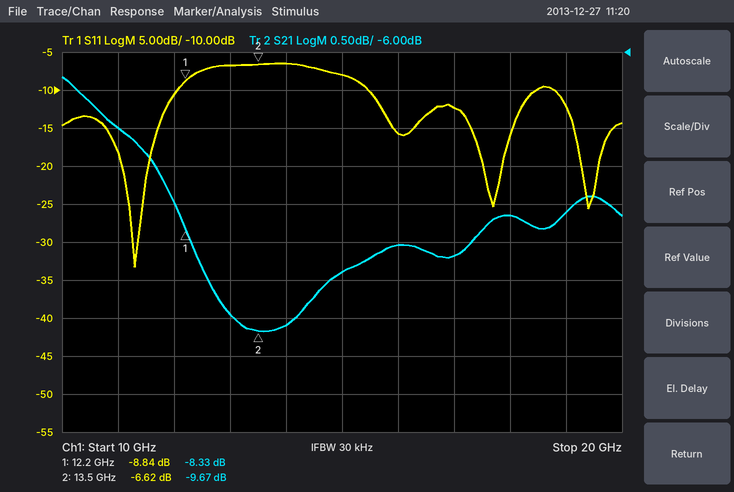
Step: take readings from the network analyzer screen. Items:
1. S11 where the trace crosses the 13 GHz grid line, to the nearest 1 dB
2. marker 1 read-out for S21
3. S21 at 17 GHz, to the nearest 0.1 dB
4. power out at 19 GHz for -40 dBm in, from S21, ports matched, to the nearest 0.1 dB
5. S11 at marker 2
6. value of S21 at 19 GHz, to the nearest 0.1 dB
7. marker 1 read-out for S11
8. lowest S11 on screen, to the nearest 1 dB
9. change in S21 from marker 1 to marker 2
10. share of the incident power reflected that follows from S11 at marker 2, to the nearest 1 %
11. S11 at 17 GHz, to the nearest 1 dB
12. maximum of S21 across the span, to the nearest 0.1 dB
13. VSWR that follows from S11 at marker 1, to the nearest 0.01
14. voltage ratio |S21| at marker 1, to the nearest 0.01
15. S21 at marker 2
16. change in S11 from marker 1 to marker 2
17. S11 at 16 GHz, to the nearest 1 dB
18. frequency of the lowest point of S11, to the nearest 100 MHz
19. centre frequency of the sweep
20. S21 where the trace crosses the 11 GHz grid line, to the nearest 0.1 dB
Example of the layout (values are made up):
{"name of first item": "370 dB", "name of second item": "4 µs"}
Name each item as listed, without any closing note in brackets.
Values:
{"S11 where the trace crosses the 13 GHz grid line, to the nearest 1 dB": "-7 dB", "marker 1 read-out for S21": "-8.33 dB", "S21 at 17 GHz, to the nearest 0.1 dB": "-8.7 dB", "power out at 19 GHz for -40 dBm in, from S21, ports matched, to the nearest 0.1 dB": "-48.1 dBm", "S11 at marker 2": "-6.62 dB", "value of S21 at 19 GHz, to the nearest 0.1 dB": "-8.1 dB", "marker 1 read-out for S11": "-8.84 dB", "lowest S11 on screen, to the nearest 1 dB": "-33 dB", "change in S21 from marker 1 to marker 2": "-1.34 dB", "share of the incident power reflected that follows from S11 at marker 2, to the nearest 1 %": "22 %", "S11 at 17 GHz, to the nearest 1 dB": "-12 dB", "maximum of S21 across the span, to the nearest 0.1 dB": "-6.3 dB", "VSWR that follows from S11 at marker 1, to the nearest 0.01": "2.13", "voltage ratio |S21| at marker 1, to the nearest 0.01": "0.38", "S21 at marker 2": "-9.67 dB", "change in S11 from marker 1 to marker 2": "2.22 dB", "S11 at 16 GHz, to the nearest 1 dB": "-16 dB", "frequency of the lowest point of S11, to the nearest 100 MHz": "11.3 GHz", "centre frequency of the sweep": "15 GHz", "S21 where the trace crosses the 11 GHz grid line, to the nearest 0.1 dB": "-7.0 dB"}
